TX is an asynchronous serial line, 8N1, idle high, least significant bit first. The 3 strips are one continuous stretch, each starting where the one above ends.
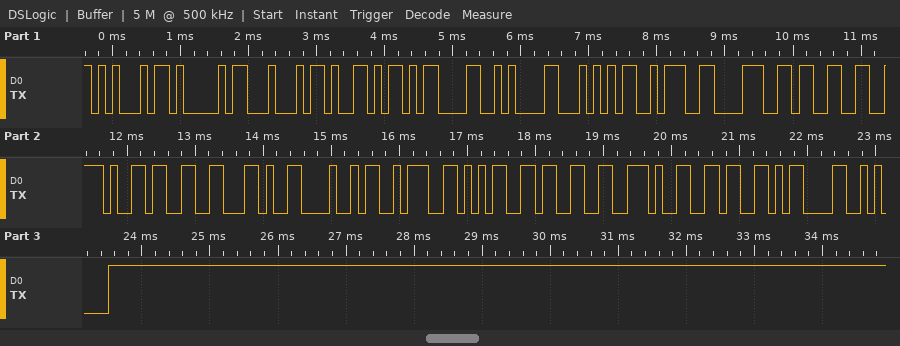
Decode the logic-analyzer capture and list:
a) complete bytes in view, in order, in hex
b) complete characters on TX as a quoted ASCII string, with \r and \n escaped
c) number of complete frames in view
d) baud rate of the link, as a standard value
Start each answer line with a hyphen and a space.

- 0x45 0x41 0x44 0x59 0x0D 0x0A 0x54 0x3A 0x38 0x33 0x2E 0x33 0x2C 0x48 0x3A 0x35 0x33 0x2E 0x36 0x0D 0x0A
- "EADY\r\nT:83.3,H:53.6\r\n"
- 21
- 9600 baud
